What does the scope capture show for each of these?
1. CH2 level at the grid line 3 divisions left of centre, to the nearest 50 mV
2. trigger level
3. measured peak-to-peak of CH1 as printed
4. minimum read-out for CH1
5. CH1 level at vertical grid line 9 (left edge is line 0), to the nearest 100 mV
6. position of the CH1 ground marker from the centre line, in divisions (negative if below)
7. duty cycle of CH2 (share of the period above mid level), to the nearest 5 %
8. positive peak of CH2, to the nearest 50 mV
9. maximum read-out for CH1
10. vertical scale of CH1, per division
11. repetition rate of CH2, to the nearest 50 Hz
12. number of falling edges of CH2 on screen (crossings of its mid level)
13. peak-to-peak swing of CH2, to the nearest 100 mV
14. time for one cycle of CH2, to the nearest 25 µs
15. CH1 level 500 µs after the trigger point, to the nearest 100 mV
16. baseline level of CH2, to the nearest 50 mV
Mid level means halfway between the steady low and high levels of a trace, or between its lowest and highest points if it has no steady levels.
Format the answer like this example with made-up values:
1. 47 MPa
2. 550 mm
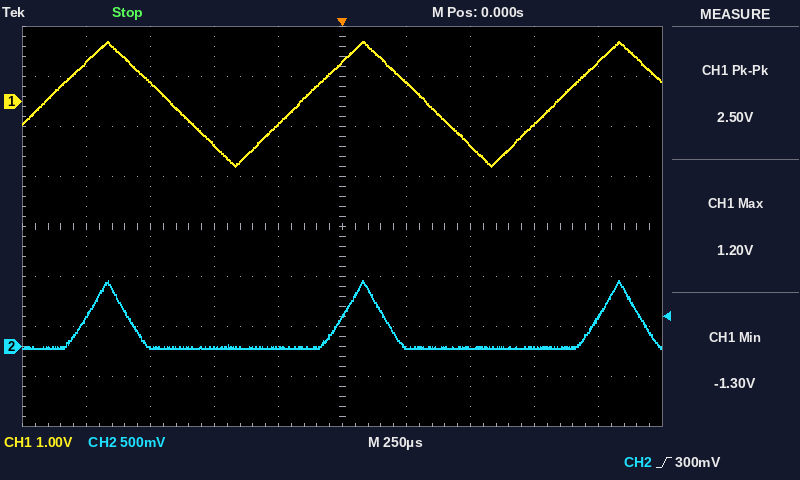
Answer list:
1. 0 mV
2. 300 mV
3. 2.50 V
4. -1.30 V
5. 800 mV
6. +2.5 div
7. 15 %
8. 650 mV
9. 1.20 V
10. 1 V
11. 1.00 kHz
12. 3
13. 700 mV
14. 1.000 ms
15. -900 mV
16. 0 mV
